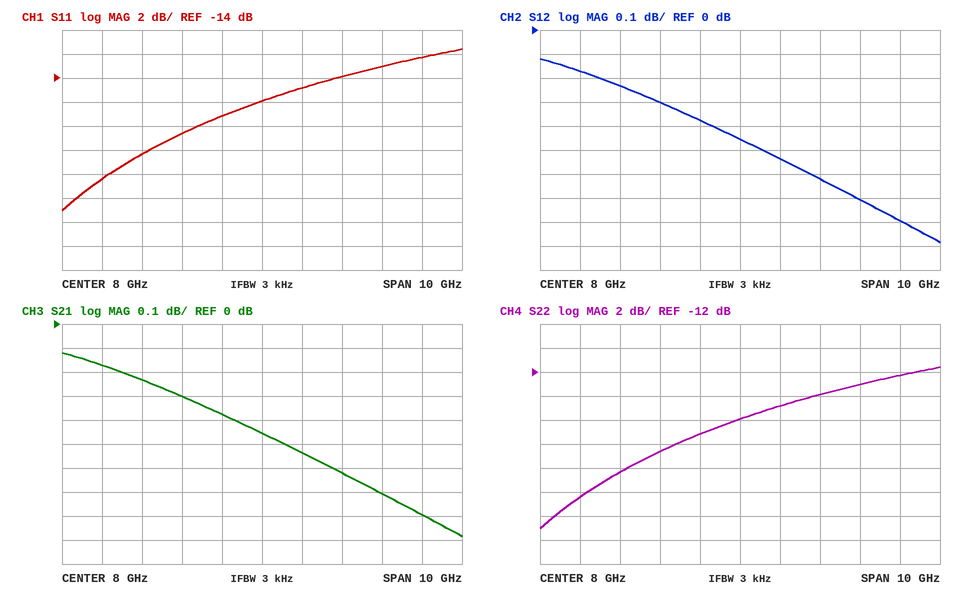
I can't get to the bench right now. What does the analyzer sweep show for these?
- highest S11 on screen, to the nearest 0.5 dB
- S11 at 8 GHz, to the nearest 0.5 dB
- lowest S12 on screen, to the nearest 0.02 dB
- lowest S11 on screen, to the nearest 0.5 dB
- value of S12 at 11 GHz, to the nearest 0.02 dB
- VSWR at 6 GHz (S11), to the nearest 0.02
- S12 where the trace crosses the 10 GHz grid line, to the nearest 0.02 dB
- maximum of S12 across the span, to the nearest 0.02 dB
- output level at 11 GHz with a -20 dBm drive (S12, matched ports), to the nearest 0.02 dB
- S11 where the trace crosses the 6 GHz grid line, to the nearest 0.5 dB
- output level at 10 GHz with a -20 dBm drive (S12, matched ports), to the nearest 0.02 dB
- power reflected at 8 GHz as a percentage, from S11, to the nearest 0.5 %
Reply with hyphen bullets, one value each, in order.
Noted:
- -11.5 dB
- -16.0 dB
- -0.88 dB
- -25.0 dB
- -0.70 dB
- 1.26
- -0.62 dB
- -0.12 dB
- -20.70 dBm
- -18.5 dB
- -20.62 dBm
- 2.5 %
